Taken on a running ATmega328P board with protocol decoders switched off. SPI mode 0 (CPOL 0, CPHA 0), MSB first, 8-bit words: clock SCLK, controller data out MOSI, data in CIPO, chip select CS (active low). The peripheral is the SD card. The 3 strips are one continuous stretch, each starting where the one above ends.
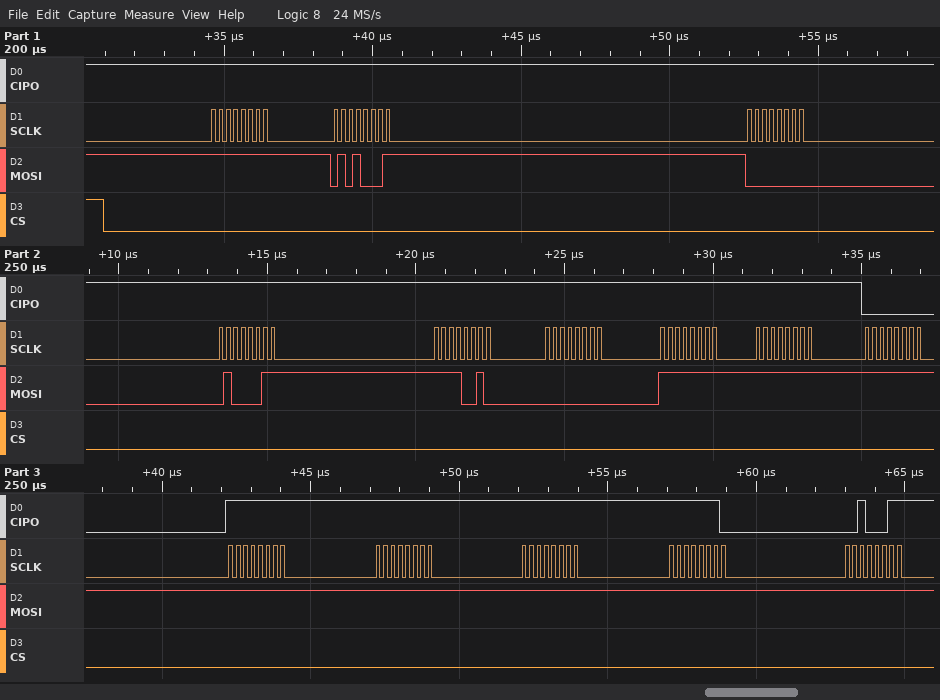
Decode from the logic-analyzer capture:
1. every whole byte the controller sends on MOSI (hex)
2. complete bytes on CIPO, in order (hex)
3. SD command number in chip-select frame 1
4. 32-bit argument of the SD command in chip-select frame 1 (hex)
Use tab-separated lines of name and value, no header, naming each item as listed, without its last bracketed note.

every whole byte the controller sends on MOSI	FF 51 00 43 F2 00 FF FF FF FF FF FF FF FF
complete bytes on CIPO, in order	FF FF FF FF FF FF FF FF 00 FF FF FF FE 23
SD command number in chip-select frame 1	CMD17
32-bit argument of the SD command in chip-select frame 1	0x0043F200
